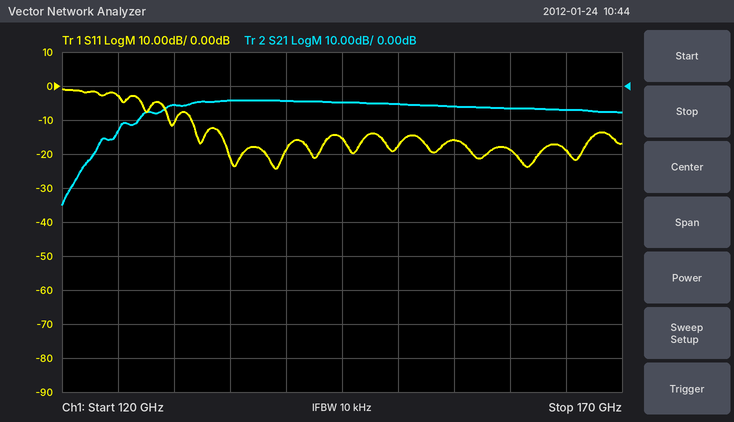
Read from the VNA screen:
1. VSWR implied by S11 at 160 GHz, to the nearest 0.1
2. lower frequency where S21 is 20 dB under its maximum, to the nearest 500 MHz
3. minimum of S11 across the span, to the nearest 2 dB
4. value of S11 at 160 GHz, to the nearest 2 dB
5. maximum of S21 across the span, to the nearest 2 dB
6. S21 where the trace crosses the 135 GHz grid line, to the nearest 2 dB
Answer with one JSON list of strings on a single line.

["1.3", "122.0 GHz", "-24 dB", "-18 dB", "-4 dB", "-4 dB"]
